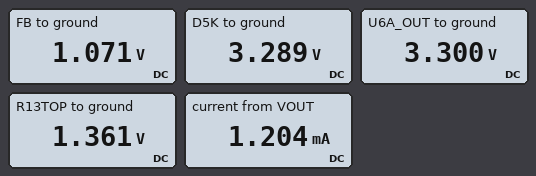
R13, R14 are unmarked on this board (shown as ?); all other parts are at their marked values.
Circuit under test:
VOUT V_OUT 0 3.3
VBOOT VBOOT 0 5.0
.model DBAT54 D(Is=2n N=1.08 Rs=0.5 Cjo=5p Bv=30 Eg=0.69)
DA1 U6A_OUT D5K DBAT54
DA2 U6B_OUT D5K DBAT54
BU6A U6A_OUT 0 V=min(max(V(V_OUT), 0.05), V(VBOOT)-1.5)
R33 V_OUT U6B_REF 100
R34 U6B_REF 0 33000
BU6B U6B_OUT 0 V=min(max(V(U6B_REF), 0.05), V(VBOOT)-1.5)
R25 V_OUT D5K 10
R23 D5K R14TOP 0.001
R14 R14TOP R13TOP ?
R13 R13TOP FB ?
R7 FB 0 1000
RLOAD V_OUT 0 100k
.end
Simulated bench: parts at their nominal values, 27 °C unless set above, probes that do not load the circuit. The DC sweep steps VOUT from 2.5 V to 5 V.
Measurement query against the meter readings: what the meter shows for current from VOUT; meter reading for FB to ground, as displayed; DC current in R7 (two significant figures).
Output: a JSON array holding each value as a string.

["1.204 mA", "1.071 V", "1.1 mA"]
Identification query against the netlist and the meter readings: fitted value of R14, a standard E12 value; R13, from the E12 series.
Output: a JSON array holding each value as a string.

["1.8 kΩ", "270 Ω"]
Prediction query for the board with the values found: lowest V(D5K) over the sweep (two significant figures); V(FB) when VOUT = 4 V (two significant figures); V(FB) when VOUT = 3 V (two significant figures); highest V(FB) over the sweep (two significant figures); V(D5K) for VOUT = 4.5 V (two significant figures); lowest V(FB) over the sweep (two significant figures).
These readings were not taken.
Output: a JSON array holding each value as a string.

["2.5 V", "1.3 V", "970 mV", "1.6 V", "4.5 V", "810 mV"]
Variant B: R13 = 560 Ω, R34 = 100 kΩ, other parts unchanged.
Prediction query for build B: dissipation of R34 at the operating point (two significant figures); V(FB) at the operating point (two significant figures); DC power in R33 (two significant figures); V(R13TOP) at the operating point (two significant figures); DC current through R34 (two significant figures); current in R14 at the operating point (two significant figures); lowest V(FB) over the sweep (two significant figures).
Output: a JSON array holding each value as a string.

["110 µW", "980 mV", "110 nW", "1.5 V", "33 µA", "980 µA", "740 mV"]
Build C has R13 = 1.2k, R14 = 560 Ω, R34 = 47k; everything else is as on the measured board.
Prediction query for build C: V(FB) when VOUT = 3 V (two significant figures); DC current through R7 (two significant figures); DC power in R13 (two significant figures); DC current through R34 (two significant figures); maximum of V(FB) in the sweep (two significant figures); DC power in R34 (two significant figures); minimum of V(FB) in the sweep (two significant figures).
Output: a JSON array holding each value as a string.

["1.1 V", "1.2 mA", "1.7 mW", "70 µA", "1.8 V", "230 µW", "900 mV"]
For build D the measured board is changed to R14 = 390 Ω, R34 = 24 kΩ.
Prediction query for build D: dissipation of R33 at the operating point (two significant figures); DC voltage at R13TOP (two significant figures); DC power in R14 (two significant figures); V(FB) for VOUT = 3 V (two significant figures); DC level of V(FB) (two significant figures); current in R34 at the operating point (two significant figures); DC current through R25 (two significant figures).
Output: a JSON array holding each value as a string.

["1.9 µW", "2.5 V", "1.5 mW", "1.8 V", "2.0 V", "140 µA", "2.0 mA"]
